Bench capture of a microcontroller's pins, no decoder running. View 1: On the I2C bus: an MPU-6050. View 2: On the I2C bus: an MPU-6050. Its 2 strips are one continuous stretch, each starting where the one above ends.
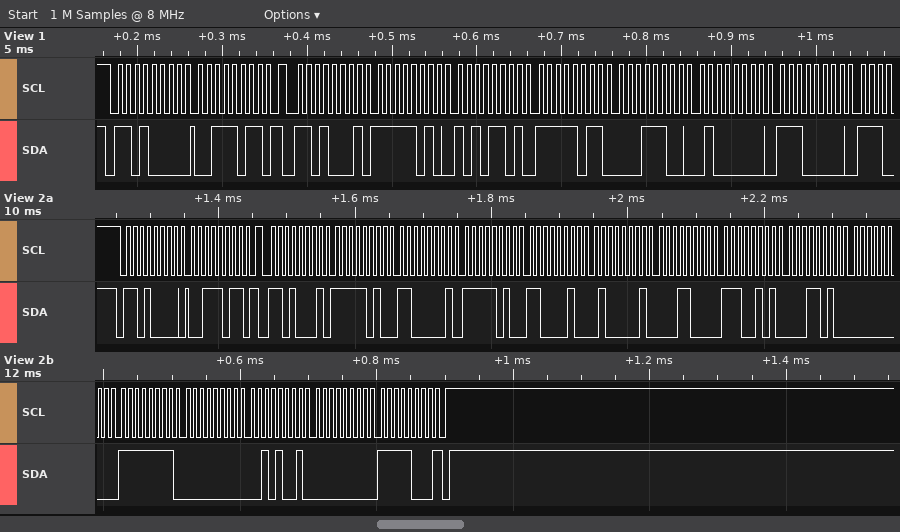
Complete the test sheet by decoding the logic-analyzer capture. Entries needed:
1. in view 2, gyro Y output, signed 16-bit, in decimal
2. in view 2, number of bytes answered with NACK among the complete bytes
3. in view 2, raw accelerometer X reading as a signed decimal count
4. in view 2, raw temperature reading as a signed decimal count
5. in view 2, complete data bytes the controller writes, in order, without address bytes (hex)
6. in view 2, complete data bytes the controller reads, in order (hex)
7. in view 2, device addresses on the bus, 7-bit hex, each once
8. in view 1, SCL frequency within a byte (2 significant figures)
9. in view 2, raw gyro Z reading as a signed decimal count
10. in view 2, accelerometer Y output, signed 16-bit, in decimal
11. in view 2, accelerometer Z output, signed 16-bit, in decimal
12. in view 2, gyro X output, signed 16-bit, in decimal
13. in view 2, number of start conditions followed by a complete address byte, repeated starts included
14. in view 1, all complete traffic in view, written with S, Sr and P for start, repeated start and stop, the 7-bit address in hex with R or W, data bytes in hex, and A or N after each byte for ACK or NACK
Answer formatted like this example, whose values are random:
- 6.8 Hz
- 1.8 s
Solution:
- 41
- 1
- -1343
- -6886
- 3B
- FA C1 FA C2 41 18 E5 1A 00 FF 00 29 00 F8
- 0x68
- 100 kHz
- 248
- -1342
- 16664
- 255
- 2
- S 68W A 3B A Sr 68R A FA A AD A FB A 1C A 40 A E0 A
